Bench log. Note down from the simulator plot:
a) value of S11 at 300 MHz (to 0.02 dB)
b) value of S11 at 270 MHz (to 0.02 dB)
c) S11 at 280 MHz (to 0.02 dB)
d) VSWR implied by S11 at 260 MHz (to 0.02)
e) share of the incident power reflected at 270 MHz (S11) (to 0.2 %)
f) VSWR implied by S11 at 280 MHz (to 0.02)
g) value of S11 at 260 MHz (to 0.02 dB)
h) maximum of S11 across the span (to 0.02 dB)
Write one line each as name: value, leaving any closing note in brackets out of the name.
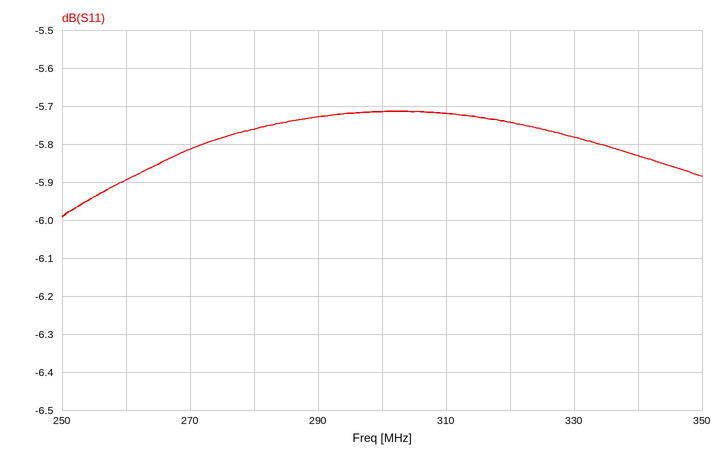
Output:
value of S11 at 300 MHz: -5.72 dB
value of S11 at 270 MHz: -5.82 dB
S11 at 280 MHz: -5.76 dB
VSWR implied by S11 at 260 MHz: 3.06
share of the incident power reflected at 270 MHz (S11): 26.2 %
VSWR implied by S11 at 280 MHz: 3.12
value of S11 at 260 MHz: -5.90 dB
maximum of S11 across the span: -5.72 dB
